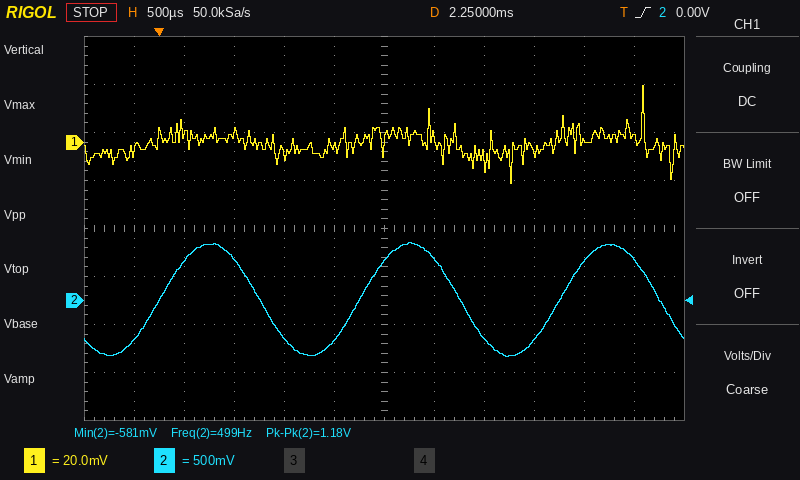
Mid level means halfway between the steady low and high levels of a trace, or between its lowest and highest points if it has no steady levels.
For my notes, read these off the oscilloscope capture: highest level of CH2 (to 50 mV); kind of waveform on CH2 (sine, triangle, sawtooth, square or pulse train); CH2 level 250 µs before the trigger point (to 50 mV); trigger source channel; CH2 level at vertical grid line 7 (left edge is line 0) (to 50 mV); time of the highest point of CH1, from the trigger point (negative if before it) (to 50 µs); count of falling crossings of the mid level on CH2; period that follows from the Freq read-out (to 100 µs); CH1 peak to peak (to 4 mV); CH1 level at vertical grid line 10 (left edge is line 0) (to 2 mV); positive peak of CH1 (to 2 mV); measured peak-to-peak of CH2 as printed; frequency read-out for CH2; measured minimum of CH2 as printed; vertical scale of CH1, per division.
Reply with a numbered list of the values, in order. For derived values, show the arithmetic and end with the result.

1. 600 mV
2. sine
3. -400 mV
4. CH2
5. 450 mV
6. +4.85 ms
7. 3
8. 1 / 499 Hz ≈ 2.0 ms
9. 40 mV
10. 0 mV
11. 24 mV
12. 1.18 V
13. 499 Hz
14. -581 mV
15. 20 mV
